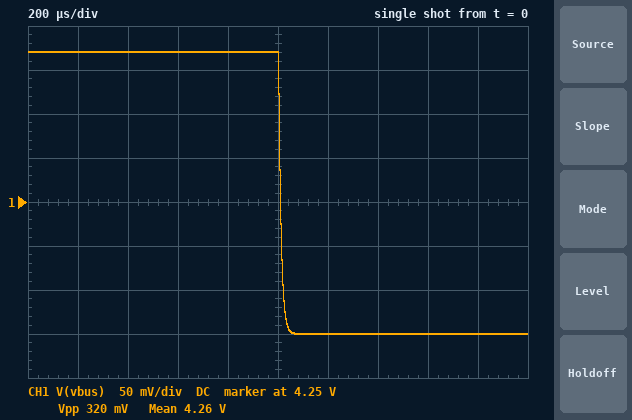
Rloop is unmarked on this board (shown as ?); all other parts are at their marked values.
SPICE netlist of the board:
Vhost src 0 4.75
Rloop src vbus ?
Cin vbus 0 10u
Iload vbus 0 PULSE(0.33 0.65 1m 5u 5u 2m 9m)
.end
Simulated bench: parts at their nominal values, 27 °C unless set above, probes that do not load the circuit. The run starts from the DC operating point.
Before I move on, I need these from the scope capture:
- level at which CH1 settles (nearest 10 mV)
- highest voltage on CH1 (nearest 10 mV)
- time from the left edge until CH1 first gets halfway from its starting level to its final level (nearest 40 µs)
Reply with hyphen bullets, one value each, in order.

- 4.10 V
- 4.42 V
- 1.00 ms
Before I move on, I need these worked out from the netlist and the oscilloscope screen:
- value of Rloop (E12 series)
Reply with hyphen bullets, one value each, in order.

- 1 Ω
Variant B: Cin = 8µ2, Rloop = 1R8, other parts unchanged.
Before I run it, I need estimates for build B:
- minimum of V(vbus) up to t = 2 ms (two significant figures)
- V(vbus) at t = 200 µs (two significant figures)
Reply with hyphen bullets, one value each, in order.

- 3.6 V
- 4.2 V
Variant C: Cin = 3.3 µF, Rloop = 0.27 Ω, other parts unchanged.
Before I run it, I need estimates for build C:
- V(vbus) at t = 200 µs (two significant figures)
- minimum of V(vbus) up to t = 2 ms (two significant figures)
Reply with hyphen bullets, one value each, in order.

- 4.7 V
- 4.6 V
